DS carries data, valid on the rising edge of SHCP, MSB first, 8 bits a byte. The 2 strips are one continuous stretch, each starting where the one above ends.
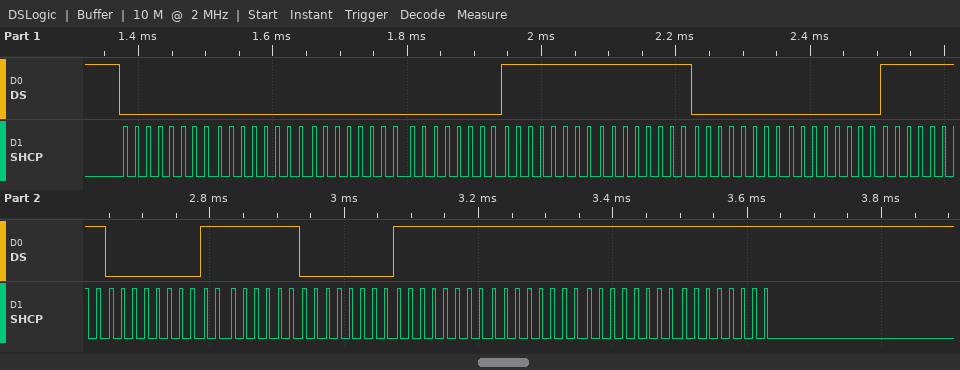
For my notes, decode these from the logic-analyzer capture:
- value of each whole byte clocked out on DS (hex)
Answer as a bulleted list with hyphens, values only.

- 0x00 0x00 0x00 0x00 0xFF 0xFF 0x00 0x00 0xFF 0x00 0xFF 0x00 0xFF 0xFF 0xFF 0xFF
